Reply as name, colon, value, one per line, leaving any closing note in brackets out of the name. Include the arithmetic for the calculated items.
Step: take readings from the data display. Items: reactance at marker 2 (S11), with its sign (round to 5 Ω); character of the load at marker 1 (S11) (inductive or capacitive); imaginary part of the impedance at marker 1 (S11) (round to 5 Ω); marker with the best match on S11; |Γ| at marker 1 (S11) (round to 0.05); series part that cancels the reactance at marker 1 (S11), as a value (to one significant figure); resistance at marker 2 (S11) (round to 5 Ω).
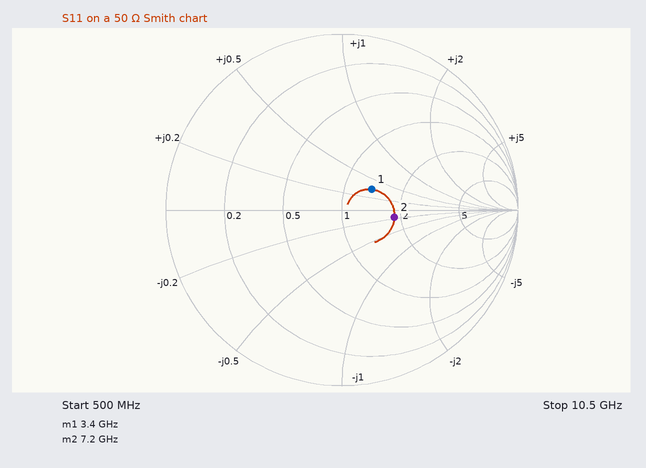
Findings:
reactance at marker 2 (S11), with its sign: -10 Ω
character of the load at marker 1 (S11): inductive
imaginary part of the impedance at marker 1 (S11): +15 Ω
marker with the best match on S11: marker 1
|Γ| at marker 1 (S11): 0.20
series part that cancels the reactance at marker 1 (S11), as a value: C = 1/(2π × 3.4 GHz × 15 Ω) ≈ 3 pF
resistance at marker 2 (S11): 90 Ω
